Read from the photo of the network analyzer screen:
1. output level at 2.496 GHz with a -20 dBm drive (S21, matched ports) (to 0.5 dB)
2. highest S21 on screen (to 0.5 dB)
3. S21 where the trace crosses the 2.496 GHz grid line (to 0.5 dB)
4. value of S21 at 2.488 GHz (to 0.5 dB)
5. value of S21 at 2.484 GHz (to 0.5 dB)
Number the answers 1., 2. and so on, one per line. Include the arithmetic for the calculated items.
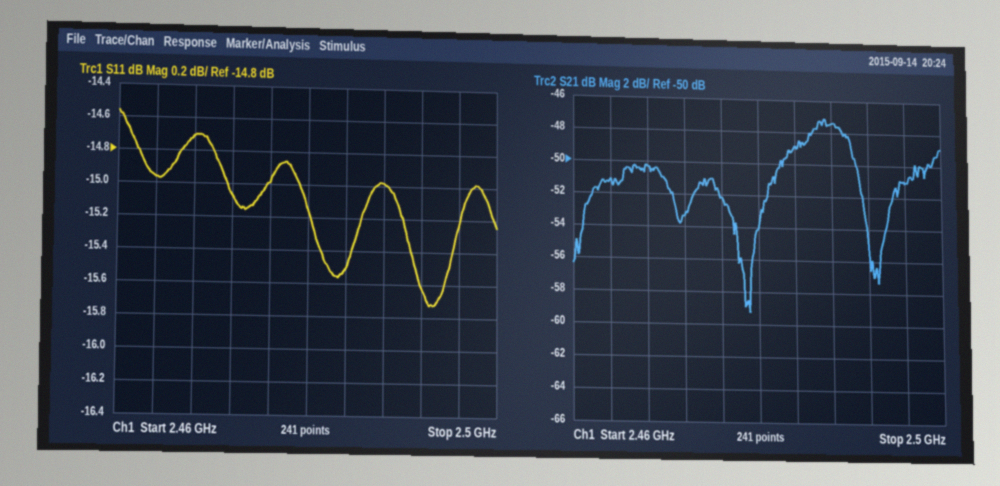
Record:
1. -20 dBm + (-51.0 dB) = -71.0 dBm
2. -47.0 dB
3. -51.0 dB
4. -47.5 dB
5. -49.0 dB
